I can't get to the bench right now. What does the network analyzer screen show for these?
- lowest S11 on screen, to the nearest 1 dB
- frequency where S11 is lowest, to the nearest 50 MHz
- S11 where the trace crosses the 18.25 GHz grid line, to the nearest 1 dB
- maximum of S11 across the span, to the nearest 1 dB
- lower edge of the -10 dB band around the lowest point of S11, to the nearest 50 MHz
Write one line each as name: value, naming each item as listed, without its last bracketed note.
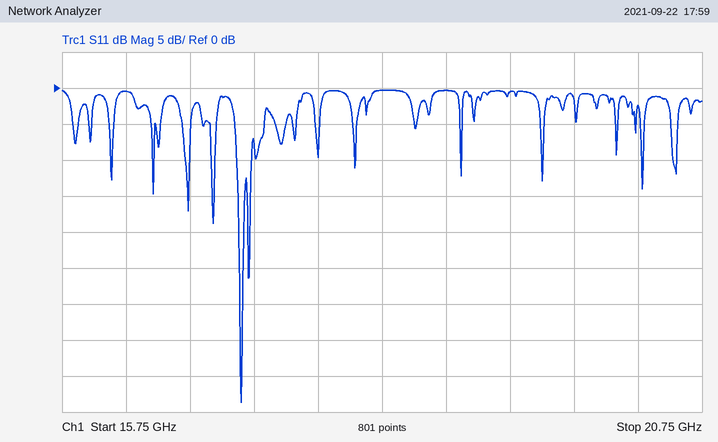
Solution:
lowest S11 on screen, to the nearest 1 dB: -44 dB
frequency where S11 is lowest, to the nearest 50 MHz: 17.15 GHz
S11 where the trace crosses the 18.25 GHz grid line, to the nearest 1 dB: 0 dB
maximum of S11 across the span, to the nearest 1 dB: 0 dB
lower edge of the -10 dB band around the lowest point of S11, to the nearest 50 MHz: 17.10 GHz
